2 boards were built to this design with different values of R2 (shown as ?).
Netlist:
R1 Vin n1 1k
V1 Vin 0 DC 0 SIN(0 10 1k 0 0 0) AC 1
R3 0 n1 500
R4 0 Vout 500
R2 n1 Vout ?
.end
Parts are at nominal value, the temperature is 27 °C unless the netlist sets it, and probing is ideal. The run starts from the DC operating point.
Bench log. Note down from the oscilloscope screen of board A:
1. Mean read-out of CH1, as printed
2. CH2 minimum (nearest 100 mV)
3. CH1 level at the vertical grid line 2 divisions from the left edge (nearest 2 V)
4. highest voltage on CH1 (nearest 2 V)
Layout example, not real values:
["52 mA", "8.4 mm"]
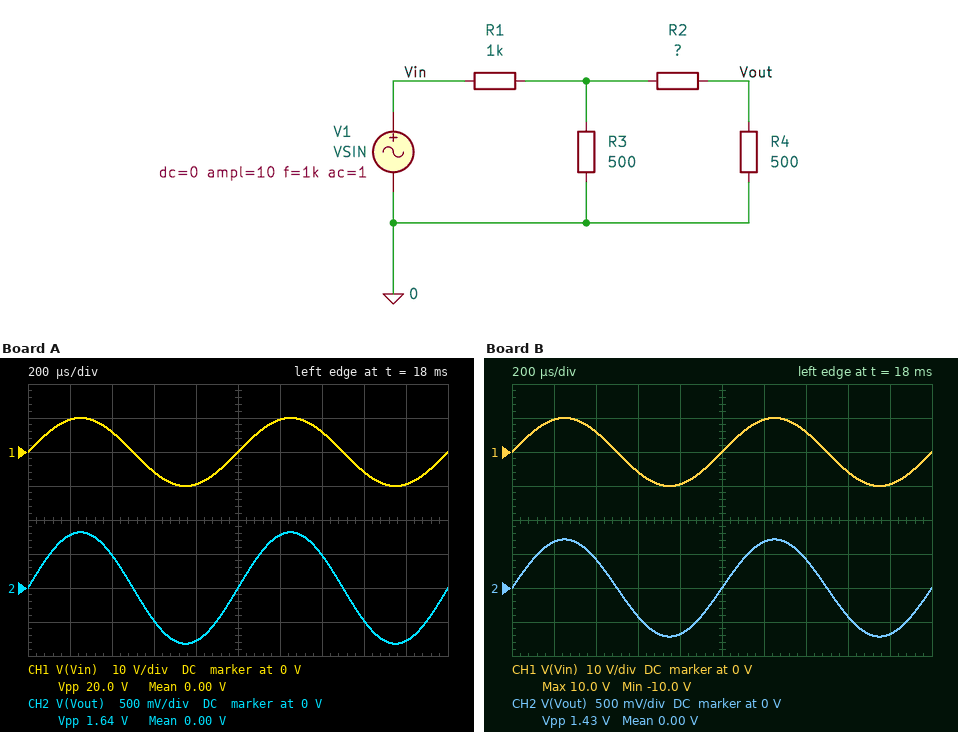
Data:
["0.00 V", "-800 mV", "6 V", "10 V"]
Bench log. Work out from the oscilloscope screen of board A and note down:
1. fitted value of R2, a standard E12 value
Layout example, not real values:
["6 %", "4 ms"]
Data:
["1.2 kΩ"]
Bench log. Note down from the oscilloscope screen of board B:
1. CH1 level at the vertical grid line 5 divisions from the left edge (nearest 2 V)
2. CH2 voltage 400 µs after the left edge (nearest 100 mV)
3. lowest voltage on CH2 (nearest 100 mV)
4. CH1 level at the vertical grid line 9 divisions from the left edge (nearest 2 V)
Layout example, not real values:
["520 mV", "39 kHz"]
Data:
["0 V", "400 mV", "-700 mV", "-10 V"]
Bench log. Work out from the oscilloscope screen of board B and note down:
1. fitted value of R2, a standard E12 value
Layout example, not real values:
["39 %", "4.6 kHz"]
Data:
["1.5 kΩ"]
